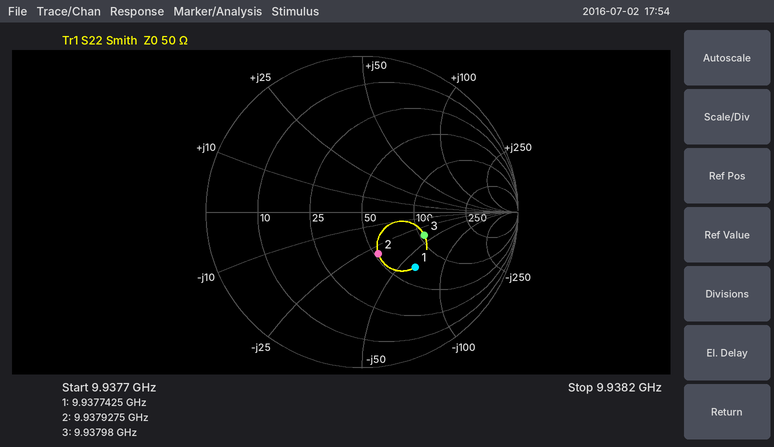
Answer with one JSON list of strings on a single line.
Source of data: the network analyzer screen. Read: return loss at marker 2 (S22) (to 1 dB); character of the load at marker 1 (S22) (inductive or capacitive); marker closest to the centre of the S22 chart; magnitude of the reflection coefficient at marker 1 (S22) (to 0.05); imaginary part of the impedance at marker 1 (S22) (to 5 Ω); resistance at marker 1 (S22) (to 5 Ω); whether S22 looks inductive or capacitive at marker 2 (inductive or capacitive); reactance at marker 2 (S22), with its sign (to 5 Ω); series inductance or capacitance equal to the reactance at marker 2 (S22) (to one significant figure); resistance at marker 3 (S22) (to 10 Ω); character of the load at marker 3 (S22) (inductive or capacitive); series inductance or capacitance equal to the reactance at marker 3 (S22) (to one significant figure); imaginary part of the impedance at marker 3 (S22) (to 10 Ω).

["11 dB", "capacitive", "marker 2", "0.50", "-65 Ω", "70 Ω", "capacitive", "-30 Ω", "500 fF", "110 Ω", "capacitive", "400 fF", "-40 Ω"]
